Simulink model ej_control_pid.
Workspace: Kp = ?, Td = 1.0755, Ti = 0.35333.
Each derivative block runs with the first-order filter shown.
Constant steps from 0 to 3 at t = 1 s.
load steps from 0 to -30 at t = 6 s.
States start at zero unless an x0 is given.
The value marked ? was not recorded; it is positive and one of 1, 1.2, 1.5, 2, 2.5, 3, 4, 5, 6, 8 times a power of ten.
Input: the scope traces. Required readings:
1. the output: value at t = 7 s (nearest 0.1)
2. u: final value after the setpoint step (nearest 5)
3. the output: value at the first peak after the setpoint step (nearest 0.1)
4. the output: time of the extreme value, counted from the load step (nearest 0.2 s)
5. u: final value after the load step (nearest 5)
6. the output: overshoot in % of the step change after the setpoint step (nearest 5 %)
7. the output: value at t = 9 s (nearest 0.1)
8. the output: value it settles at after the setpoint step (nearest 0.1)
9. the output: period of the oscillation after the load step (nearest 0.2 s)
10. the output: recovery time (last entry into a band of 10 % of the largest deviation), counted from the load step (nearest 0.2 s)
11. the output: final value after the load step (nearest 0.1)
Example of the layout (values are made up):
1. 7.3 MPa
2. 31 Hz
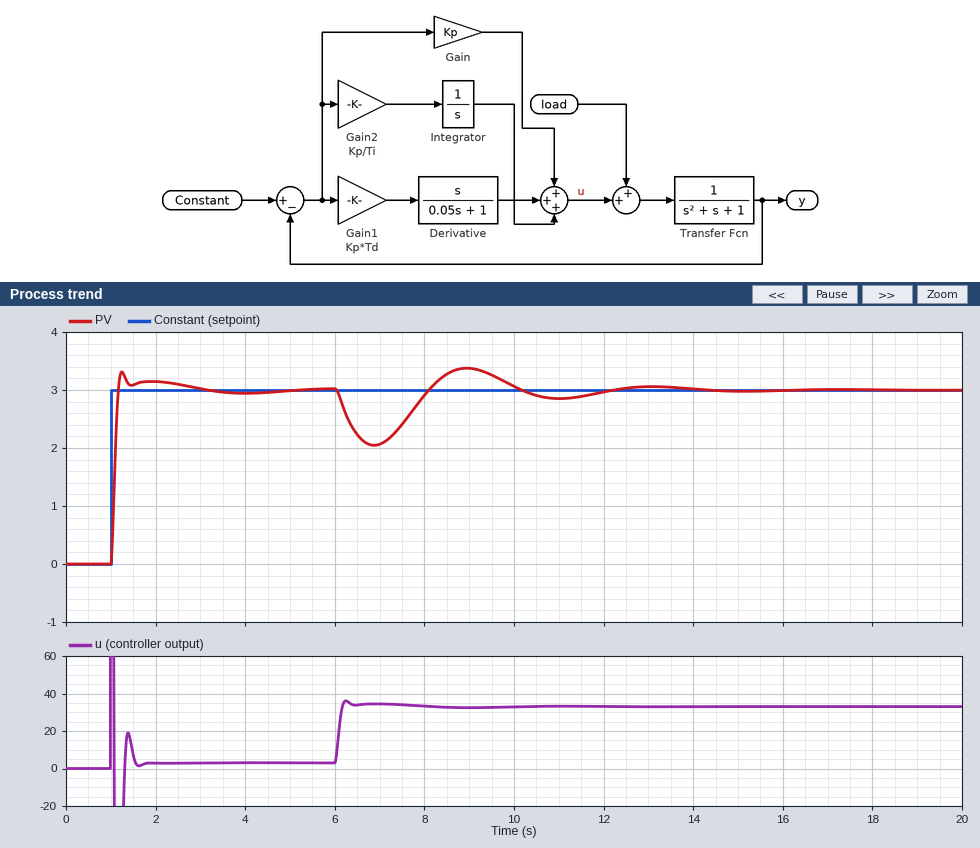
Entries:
1. 2.1
2. 5
3. 3.3
4. 0.8 s
5. 35
6. 10 %
7. 3.4
8. 3.0
9. 4.2 s
10. 5.6 s
11. 3.0
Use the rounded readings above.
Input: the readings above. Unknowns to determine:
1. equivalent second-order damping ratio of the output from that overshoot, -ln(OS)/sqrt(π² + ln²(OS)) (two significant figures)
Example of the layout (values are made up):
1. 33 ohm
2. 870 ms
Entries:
1. 0.59
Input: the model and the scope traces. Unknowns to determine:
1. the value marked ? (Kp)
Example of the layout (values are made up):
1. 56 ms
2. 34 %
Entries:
1. 12
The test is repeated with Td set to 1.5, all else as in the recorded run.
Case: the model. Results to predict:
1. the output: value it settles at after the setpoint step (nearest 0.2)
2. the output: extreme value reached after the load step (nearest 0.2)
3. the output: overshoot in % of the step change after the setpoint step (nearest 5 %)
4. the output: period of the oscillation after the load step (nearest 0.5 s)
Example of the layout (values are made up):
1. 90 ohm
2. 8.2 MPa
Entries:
1. 3.0
2. 2.2
3. 15 %
4. 5.0 s
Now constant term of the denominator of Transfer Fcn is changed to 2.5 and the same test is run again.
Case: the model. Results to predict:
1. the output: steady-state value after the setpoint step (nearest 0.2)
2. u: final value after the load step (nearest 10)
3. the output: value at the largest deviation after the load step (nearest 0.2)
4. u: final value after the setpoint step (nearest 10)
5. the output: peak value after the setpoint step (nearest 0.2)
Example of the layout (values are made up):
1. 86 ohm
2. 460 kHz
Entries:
1. 3.0
2. 40
3. 2.0
4. 10
5. 3.2
